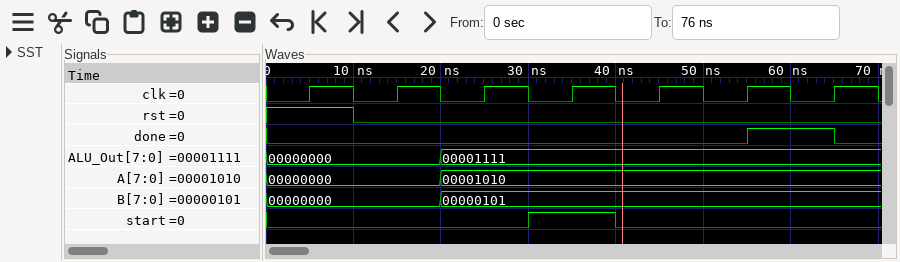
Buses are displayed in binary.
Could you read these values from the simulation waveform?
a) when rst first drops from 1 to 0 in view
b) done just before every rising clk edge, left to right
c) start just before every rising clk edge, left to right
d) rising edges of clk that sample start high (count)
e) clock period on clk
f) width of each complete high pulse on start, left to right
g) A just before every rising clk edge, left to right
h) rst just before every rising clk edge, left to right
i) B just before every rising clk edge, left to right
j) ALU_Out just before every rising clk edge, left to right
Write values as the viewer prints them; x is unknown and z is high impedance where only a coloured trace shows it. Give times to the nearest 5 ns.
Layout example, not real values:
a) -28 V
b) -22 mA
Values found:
a) 10 ns
b) 0 0 0 0 0 0 1
c) 0 0 0 1 0 0 0
d) 1
e) 10 ns
f) 10 ns
g) 00000000, 00000000, 00001010, 00001010, 00001010, 00001010, 00001010
h) 1 0 0 0 0 0 0
i) 00000000, 00000000, 00000101, 00000101, 00000101, 00000101, 00000101
j) 00000000, 00000000, 00001111, 00001111, 00001111, 00001111, 00001111
